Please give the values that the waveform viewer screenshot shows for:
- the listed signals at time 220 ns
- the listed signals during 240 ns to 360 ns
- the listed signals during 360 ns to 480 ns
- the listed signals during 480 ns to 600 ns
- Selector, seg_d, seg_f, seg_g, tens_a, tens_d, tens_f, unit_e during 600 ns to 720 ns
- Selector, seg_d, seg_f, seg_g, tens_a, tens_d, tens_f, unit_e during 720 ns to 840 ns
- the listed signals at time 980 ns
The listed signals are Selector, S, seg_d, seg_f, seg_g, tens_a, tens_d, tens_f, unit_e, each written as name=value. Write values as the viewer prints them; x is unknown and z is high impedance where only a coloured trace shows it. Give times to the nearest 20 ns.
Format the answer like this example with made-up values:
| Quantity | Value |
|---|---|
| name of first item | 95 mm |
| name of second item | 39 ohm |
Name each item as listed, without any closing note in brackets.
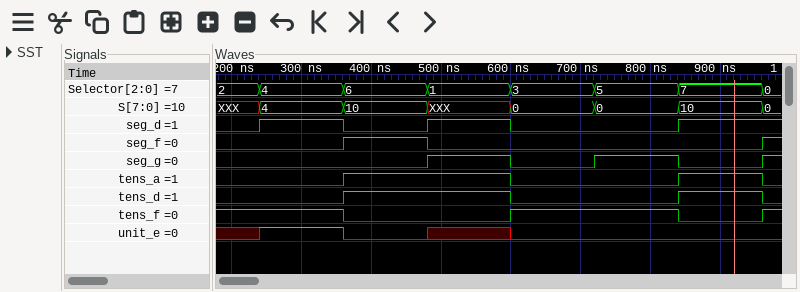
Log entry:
| Quantity | Value |
|---|---|
| the listed signals at time 220 ns | Selector=2, S=XXX, seg_d=0, seg_f=0, seg_g=0, tens_a=0, tens_d=0, tens_f=1, unit_e=x |
| the listed signals during 240 ns to 360 ns | Selector=4, S=4, seg_d=1, seg_f=0, seg_g=0, tens_a=0, tens_d=0, tens_f=1, unit_e=1 |
| the listed signals during 360 ns to 480 ns | Selector=6, S=10, seg_d=0, seg_f=1, seg_g=0, tens_a=1, tens_d=1, tens_f=0, unit_e=0 |
| the listed signals during 480 ns to 600 ns | Selector=1, S=XXX, seg_d=1, seg_f=0, seg_g=1, tens_a=1, tens_d=1, tens_f=0, unit_e=x |
| Selector, seg_d, seg_f, seg_g, tens_a, tens_d, tens_f, unit_e during 600 ns to 720 ns | Selector=3, seg_d=0, seg_f=0, seg_g=0, tens_a=0, tens_d=0, tens_f=1, unit_e=0 |
| Selector, seg_d, seg_f, seg_g, tens_a, tens_d, tens_f, unit_e during 720 ns to 840 ns | Selector=5, seg_d=0, seg_f=0, seg_g=1, tens_a=0, tens_d=0, tens_f=1, unit_e=0 |
| the listed signals at time 980 ns | Selector=0, S=0, seg_d=1, seg_f=1, seg_g=1, tens_a=0, tens_d=0, tens_f=1, unit_e=0 |
